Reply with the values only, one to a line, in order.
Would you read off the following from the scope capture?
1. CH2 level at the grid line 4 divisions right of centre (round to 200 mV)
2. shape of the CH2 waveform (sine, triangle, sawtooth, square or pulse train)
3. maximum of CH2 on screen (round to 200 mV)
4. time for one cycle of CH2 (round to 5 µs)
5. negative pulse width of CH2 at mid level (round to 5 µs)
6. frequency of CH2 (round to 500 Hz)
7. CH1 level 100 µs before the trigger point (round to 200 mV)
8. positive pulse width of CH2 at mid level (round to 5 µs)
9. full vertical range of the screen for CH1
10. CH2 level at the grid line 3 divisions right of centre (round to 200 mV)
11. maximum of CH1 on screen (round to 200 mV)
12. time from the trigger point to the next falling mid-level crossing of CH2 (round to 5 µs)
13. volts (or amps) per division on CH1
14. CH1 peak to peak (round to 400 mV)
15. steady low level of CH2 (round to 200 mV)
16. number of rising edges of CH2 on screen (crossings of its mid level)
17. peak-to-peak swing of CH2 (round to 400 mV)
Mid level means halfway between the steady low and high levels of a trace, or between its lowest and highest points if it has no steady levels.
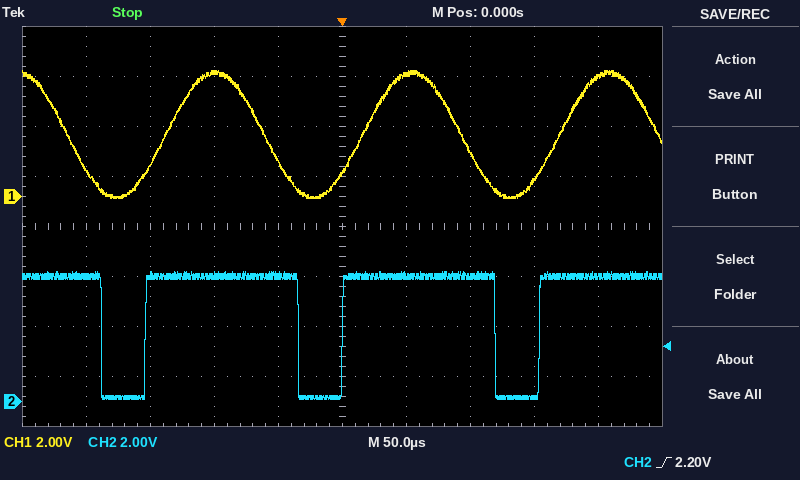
5.0 V
pulse train
5.2 V
155 µs
35 µs
6.5 kHz
5.0 V
120 µs
16 V
200 mV
5.0 V
120 µs
2 V
5.2 V
200 mV
3
5.2 V
